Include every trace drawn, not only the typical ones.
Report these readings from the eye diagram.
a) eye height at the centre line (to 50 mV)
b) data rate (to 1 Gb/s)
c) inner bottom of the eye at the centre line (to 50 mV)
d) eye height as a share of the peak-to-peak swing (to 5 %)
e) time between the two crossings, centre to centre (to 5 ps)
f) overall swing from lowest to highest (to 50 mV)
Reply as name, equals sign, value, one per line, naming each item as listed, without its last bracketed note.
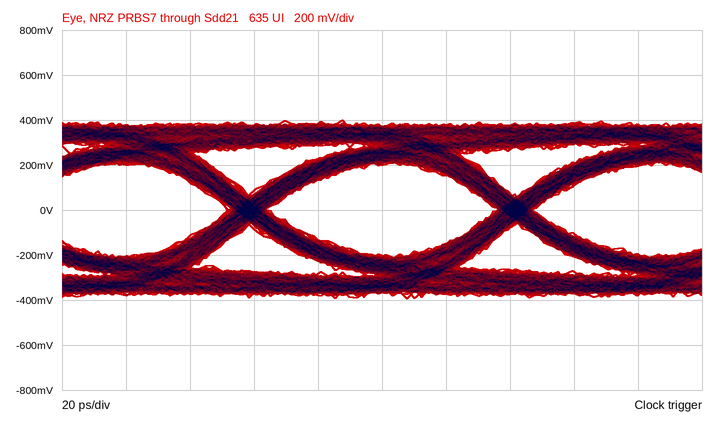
eye height at the centre line = 400 mV
data rate = 12 Gb/s
inner bottom of the eye at the centre line = -200 mV
eye height as a share of the peak-to-peak swing = 50 %
time between the two crossings, centre to centre = 85 ps
overall swing from lowest to highest = 800 mV
